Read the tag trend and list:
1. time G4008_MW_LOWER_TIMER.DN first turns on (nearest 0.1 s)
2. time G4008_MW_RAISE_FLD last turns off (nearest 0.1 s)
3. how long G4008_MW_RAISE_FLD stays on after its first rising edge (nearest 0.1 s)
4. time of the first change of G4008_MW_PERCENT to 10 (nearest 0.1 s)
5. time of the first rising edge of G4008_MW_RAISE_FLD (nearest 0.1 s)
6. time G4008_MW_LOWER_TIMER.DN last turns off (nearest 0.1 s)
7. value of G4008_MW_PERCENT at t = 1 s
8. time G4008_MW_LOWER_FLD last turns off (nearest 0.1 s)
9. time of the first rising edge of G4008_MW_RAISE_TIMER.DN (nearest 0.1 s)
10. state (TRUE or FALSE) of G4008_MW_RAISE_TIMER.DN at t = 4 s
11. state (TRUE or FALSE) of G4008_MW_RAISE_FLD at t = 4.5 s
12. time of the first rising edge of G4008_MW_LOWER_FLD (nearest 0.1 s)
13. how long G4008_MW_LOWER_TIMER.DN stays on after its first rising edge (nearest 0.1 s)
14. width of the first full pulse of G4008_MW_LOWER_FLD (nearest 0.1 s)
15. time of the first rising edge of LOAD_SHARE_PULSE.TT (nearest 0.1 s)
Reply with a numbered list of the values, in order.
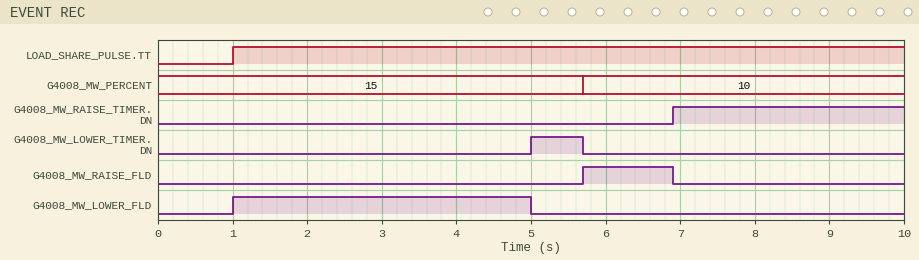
1. 5.0 s
2. 6.9 s
3. 1.2 s
4. 5.7 s
5. 5.7 s
6. 5.7 s
7. 15
8. 5.0 s
9. 6.9 s
10. FALSE
11. FALSE
12. 1.0 s
13. 0.7 s
14. 4.0 s
15. 1.0 s
